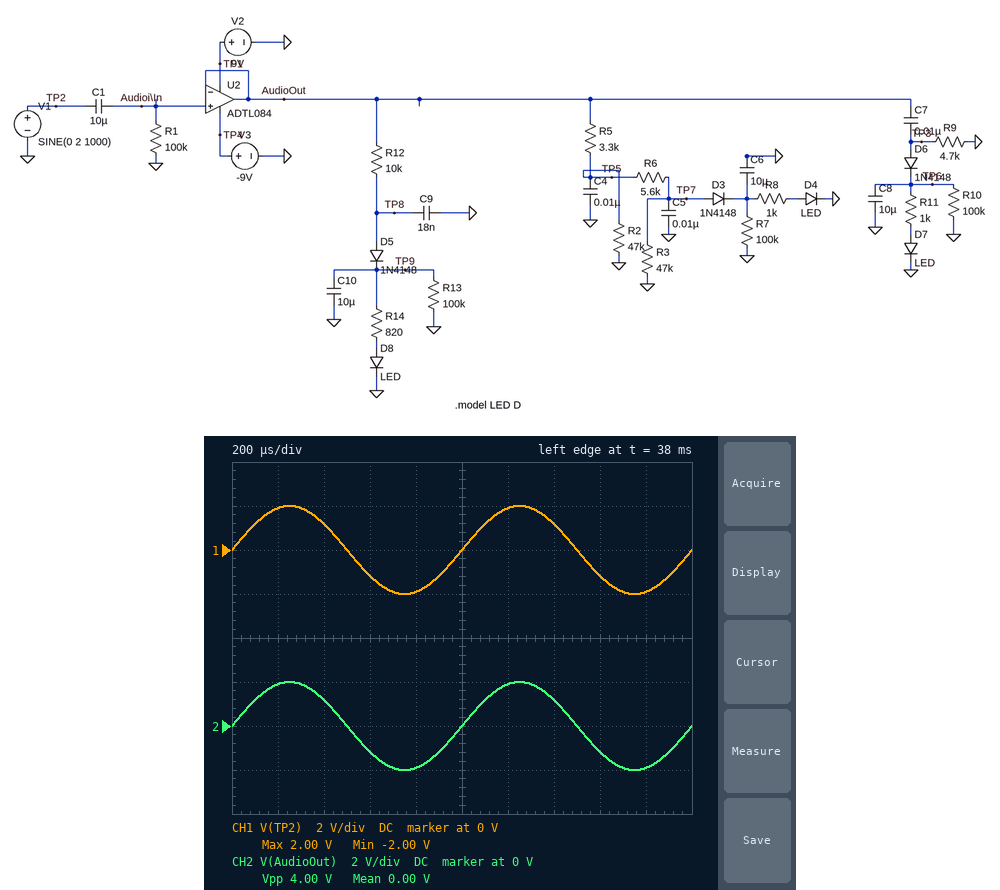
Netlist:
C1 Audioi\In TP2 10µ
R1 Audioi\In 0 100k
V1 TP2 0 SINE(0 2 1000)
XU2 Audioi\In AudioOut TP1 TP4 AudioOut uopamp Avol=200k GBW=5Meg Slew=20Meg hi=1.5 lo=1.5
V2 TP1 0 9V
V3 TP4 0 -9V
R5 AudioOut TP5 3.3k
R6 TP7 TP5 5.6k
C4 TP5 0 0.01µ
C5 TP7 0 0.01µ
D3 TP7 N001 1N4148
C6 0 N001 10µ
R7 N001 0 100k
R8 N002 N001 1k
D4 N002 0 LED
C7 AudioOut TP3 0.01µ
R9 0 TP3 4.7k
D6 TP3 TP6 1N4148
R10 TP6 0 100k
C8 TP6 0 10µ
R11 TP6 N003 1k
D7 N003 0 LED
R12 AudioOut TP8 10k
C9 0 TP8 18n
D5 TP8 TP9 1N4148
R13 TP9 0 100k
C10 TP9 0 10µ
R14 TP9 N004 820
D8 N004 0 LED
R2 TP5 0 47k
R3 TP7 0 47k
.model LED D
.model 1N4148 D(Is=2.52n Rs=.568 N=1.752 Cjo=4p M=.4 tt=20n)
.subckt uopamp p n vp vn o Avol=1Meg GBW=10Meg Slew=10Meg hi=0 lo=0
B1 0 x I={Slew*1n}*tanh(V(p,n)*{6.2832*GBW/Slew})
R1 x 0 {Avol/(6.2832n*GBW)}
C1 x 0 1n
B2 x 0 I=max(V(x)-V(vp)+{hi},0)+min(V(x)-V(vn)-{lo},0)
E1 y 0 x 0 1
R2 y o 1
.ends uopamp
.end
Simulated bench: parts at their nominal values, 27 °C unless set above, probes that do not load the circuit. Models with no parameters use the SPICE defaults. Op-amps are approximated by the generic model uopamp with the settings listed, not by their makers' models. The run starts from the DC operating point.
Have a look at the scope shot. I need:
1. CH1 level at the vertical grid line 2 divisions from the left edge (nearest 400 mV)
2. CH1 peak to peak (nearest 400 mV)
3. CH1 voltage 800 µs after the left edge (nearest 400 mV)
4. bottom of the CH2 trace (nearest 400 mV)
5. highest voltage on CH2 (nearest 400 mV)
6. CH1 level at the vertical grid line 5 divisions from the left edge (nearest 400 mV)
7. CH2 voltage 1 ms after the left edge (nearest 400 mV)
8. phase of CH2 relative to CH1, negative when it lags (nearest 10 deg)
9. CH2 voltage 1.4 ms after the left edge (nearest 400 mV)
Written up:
1.2 V
4.0 V
-2.0 V
-2.0 V
2.0 V
0 V
0 V
0 deg
1.2 V
